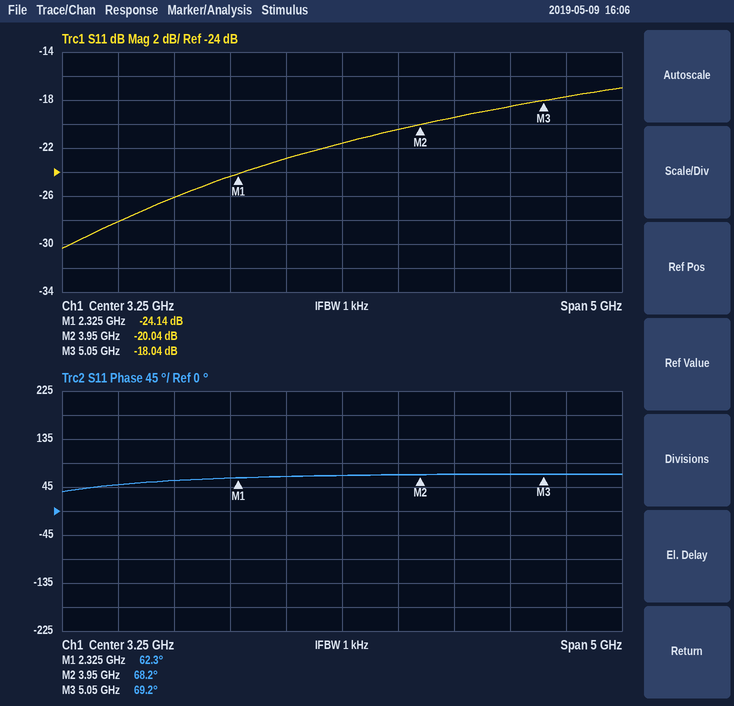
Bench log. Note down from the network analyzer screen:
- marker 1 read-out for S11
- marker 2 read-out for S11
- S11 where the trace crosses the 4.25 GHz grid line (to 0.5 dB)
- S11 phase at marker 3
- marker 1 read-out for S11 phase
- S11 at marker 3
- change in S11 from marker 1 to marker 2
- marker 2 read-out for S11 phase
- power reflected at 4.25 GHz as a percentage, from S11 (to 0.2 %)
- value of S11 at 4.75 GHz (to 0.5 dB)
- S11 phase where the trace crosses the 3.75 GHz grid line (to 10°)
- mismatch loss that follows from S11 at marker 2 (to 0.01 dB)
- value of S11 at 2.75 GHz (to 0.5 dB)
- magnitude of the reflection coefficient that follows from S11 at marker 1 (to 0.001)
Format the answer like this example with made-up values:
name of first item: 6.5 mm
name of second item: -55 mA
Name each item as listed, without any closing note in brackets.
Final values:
marker 1 read-out for S11: -24.14 dB
marker 2 read-out for S11: -20.04 dB
S11 where the trace crosses the 4.25 GHz grid line: -19.5 dB
S11 phase at marker 3: 69.2°
marker 1 read-out for S11 phase: 62.3°
S11 at marker 3: -18.04 dB
change in S11 from marker 1 to marker 2: 4.10 dB
marker 2 read-out for S11 phase: 68.2°
power reflected at 4.25 GHz as a percentage, from S11: 1.2 %
value of S11 at 4.75 GHz: -18.5 dB
S11 phase where the trace crosses the 3.75 GHz grid line: 70°
mismatch loss that follows from S11 at marker 2: 0.04 dB
value of S11 at 2.75 GHz: -23.0 dB
magnitude of the reflection coefficient that follows from S11 at marker 1: 0.062
